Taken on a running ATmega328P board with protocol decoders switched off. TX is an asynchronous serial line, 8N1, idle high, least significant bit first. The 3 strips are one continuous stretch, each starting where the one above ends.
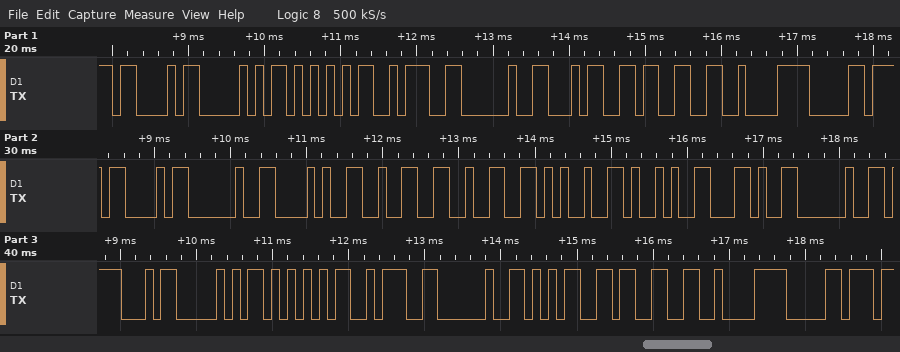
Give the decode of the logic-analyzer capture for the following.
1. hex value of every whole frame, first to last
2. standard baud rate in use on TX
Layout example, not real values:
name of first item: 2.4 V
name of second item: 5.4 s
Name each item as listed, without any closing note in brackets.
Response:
hex value of every whole frame, first to last: 43 50 55 3A 20 34 33 C2 B0 43 20 28 32 32 25 29 2C 20 47 50 55 3A 20 35 33 C2 B0
standard baud rate in use on TX: 9600 baud
